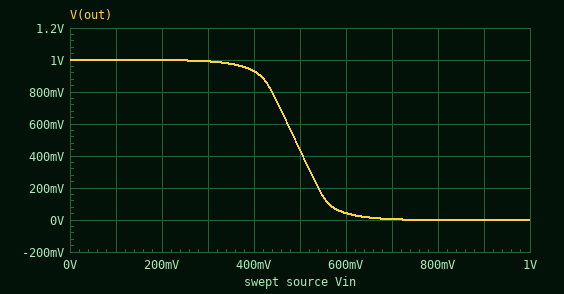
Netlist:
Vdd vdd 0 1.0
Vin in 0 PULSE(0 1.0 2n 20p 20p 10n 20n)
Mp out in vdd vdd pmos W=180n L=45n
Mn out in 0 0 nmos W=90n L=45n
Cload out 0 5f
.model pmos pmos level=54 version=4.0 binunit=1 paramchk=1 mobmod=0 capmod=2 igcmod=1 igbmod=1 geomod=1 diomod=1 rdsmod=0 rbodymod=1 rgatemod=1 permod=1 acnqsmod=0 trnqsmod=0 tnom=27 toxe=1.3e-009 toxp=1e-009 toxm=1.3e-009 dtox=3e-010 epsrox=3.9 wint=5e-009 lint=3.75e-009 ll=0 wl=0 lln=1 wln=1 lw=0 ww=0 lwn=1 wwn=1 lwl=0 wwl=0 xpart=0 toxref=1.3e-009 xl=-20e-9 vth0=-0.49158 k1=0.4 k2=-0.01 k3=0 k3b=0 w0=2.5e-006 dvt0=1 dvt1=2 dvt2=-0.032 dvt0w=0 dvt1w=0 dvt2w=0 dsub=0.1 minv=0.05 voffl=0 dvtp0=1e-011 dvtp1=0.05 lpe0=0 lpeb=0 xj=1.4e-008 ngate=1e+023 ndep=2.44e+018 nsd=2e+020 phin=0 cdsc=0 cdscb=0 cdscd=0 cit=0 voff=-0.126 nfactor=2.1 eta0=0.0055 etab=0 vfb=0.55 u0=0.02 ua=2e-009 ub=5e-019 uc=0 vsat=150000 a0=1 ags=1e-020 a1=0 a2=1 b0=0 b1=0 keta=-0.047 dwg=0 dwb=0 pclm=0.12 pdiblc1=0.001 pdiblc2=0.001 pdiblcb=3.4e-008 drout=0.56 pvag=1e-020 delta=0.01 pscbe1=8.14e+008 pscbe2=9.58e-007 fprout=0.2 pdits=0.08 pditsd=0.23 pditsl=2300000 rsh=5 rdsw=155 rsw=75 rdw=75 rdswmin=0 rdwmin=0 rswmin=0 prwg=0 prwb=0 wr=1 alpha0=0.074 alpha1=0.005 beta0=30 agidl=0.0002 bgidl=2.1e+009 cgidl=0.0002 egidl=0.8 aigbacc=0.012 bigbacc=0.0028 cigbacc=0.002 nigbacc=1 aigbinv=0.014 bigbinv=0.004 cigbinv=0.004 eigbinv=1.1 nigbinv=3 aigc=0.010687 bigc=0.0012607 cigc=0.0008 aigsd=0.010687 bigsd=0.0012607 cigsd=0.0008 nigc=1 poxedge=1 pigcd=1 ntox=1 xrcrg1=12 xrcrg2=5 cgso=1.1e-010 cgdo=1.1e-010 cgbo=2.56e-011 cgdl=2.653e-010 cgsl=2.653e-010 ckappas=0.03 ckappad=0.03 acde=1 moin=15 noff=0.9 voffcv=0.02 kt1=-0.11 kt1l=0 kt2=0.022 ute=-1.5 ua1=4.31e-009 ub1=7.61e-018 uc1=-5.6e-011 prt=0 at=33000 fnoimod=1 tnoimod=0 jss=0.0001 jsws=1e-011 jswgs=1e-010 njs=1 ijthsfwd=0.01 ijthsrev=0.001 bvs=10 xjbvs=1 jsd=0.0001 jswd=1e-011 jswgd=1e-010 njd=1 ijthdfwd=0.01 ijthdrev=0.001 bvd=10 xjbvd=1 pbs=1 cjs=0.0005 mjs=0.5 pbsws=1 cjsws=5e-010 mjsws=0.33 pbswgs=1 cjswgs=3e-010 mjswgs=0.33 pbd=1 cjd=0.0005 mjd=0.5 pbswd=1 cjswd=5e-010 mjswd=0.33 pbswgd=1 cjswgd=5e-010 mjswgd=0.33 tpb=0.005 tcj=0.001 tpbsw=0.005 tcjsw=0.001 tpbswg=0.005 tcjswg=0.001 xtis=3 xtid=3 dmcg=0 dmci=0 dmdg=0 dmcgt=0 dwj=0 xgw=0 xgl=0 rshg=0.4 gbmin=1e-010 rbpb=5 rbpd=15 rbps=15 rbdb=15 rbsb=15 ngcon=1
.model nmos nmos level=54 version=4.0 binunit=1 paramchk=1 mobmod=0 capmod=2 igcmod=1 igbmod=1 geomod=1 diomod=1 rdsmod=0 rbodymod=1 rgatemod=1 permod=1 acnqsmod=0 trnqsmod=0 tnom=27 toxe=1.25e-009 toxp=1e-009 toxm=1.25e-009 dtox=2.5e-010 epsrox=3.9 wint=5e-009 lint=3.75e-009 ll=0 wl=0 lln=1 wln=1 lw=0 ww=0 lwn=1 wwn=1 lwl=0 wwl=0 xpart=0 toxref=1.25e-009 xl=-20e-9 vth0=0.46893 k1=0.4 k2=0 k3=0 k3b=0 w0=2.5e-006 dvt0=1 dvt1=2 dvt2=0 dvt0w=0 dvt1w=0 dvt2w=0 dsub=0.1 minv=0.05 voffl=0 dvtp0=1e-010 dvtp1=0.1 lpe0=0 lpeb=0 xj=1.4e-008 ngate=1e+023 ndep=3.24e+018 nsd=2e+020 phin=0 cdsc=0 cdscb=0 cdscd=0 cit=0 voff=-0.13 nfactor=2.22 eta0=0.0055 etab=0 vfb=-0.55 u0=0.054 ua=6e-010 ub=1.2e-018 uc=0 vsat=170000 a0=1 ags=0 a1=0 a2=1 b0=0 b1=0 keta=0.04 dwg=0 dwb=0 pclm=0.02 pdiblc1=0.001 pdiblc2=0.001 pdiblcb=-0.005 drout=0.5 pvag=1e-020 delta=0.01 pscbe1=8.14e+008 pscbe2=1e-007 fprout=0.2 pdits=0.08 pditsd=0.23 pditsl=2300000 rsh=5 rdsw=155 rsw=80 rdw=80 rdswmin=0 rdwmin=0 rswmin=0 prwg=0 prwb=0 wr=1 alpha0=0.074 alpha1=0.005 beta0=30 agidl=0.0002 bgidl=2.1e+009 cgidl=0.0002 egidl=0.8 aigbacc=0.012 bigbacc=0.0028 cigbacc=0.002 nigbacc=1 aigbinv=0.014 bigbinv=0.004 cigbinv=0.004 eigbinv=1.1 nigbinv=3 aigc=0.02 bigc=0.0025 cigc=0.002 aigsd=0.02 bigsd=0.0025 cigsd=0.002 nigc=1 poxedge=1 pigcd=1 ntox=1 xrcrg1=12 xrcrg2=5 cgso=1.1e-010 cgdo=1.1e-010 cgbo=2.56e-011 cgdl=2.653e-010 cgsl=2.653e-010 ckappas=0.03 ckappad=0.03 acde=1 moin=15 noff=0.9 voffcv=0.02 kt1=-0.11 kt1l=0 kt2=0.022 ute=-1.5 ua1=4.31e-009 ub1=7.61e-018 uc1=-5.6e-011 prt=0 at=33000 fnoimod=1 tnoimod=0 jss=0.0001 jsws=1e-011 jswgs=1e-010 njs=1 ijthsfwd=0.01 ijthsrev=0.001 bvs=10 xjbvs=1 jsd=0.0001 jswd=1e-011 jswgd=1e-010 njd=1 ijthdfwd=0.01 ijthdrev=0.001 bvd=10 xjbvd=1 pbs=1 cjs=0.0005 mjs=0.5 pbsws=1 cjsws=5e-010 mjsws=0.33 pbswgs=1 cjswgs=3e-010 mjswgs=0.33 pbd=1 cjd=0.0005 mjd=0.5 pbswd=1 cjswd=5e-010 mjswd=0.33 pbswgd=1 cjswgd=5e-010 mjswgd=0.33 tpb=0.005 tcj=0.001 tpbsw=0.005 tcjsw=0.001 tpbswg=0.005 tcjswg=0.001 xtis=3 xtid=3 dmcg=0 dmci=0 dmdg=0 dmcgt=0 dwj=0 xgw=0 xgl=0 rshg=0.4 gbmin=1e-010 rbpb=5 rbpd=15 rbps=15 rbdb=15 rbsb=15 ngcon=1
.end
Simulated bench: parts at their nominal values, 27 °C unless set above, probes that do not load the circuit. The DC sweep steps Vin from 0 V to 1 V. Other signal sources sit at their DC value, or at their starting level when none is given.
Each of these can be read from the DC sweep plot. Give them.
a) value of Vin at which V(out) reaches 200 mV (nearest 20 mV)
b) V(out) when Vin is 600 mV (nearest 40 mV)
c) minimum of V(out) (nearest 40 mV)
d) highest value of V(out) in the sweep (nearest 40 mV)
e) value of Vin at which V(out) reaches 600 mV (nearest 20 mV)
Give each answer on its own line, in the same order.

540 mV
40 mV
0 V
1.00 V
480 mV
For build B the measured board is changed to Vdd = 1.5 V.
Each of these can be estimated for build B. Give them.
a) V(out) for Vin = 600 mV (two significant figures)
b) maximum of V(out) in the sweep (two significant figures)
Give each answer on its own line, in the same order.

1.3 V
1.5 V
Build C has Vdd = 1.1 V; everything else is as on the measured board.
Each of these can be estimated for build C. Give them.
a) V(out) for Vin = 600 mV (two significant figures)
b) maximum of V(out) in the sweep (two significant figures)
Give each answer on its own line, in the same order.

240 mV
1.1 V
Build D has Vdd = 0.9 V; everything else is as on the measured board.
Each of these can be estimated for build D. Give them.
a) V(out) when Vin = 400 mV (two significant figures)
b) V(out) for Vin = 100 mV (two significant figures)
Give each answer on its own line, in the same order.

670 mV
900 mV
